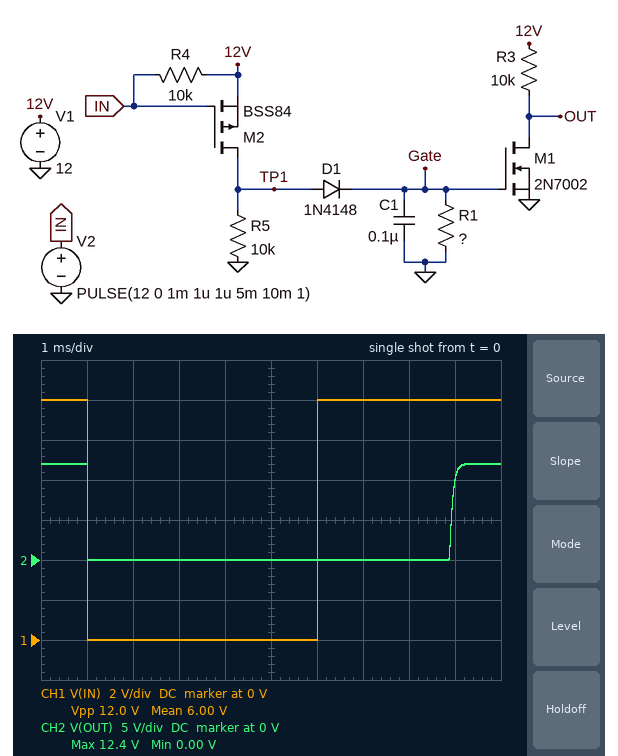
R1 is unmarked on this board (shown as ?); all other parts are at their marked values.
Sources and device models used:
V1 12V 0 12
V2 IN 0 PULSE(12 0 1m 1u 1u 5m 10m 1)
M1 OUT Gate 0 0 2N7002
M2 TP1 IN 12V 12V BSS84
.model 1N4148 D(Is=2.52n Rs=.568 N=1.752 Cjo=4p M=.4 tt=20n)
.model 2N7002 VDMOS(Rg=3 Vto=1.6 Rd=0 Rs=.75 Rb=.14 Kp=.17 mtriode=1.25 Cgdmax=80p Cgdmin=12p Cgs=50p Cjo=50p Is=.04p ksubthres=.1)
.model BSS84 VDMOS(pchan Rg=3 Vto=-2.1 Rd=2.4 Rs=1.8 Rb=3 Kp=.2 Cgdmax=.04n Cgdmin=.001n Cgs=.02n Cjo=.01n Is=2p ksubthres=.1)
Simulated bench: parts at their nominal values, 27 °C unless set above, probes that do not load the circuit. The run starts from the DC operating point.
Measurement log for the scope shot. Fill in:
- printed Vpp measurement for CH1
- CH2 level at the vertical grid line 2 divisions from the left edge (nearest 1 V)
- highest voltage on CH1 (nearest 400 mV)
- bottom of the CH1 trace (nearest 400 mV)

12.0 V
0 V
12.0 V
0 V
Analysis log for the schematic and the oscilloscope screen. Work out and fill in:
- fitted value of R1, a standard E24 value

15 kΩ
